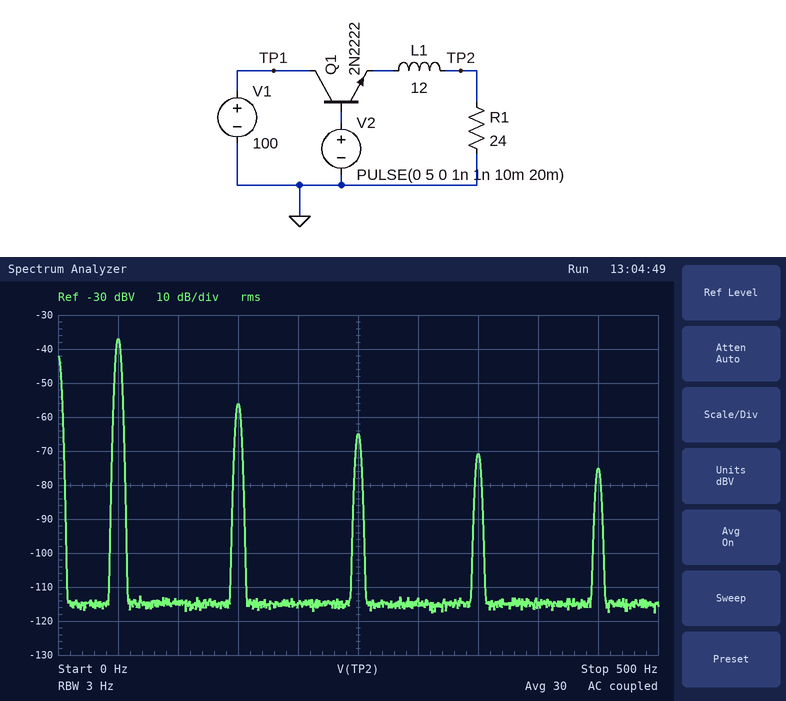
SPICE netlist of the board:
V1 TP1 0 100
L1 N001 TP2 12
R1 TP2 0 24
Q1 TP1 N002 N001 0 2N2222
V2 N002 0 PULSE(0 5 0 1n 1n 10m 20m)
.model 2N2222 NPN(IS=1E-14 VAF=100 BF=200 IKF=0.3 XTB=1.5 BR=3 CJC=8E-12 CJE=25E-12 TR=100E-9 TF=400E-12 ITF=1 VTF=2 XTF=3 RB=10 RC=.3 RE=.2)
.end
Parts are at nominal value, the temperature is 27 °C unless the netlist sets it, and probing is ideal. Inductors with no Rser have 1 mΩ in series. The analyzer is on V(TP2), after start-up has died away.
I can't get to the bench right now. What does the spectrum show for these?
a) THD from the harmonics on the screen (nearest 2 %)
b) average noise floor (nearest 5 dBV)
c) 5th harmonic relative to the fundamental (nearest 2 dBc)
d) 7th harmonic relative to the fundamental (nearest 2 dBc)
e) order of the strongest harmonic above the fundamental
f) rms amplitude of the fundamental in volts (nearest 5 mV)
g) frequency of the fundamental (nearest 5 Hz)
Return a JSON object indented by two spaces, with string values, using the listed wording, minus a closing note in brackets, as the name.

{
  "THD from the harmonics on the screen": "12 %",
  "average noise floor": "-115 dBV",
  "5th harmonic relative to the fundamental": "-28 dBc",
  "7th harmonic relative to the fundamental": "-34 dBc",
  "order of the strongest harmonic above the fundamental": "3",
  "rms amplitude of the fundamental in volts": "15 mV",
  "frequency of the fundamental": "50 Hz"
}
